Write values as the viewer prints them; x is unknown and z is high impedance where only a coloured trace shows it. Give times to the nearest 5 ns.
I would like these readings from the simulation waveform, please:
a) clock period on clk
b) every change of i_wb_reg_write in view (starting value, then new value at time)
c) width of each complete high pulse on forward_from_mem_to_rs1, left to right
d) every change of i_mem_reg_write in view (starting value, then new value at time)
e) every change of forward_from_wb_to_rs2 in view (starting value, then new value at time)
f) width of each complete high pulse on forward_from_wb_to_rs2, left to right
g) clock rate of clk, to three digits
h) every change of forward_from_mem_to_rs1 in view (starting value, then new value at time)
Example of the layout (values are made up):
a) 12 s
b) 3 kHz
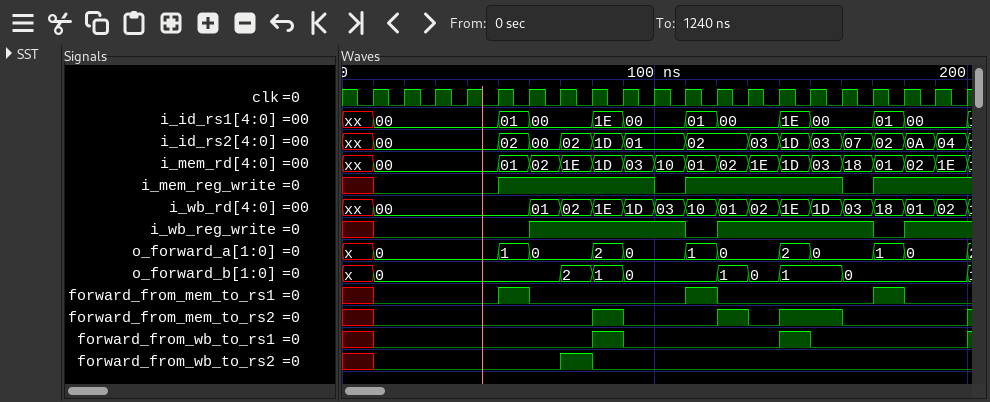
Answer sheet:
a) 10 ns
b) x, 0 at 10 ns, 1 at 60 ns, 0 at 110 ns, 1 at 120 ns, 0 at 170 ns, 1 at 180 ns
c) 10 ns, 10 ns, 10 ns
d) x, 0 at 10 ns, 1 at 50 ns, 0 at 100 ns, 1 at 110 ns, 0 at 160 ns, 1 at 170 ns
e) x, 0 at 10 ns, 1 at 70 ns, 0 at 80 ns
f) 10 ns
g) 100 MHz
h) x, 0 at 10 ns, 1 at 50 ns, 0 at 60 ns, 1 at 110 ns, 0 at 120 ns, 1 at 170 ns, 0 at 180 ns
